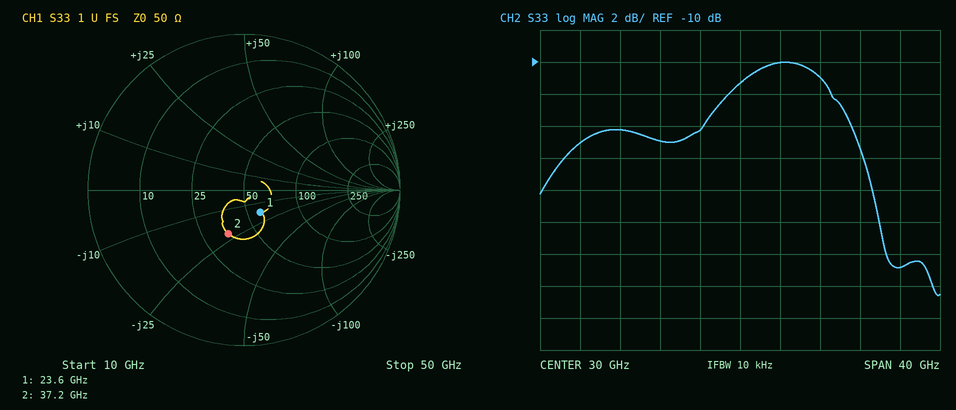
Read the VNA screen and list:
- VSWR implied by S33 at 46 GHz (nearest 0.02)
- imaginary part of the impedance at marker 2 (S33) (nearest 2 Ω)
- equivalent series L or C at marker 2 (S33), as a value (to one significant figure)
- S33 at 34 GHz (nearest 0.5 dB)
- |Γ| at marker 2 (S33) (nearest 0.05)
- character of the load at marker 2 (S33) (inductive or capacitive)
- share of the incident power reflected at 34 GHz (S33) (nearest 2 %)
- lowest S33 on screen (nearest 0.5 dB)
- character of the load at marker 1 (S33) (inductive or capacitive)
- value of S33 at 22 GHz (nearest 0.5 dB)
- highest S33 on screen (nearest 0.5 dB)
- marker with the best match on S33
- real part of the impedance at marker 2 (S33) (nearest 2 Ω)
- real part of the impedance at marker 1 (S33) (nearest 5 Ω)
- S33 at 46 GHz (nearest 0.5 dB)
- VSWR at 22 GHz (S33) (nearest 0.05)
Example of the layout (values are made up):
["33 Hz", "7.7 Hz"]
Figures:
["1.16", "-22 Ω", "200 fF", "-10.0 dB", "0.30", "capacitive", "10 %", "-24.5 dB", "capacitive", "-15.0 dB", "-10.0 dB", "marker 1", "36 Ω", "60 Ω", "-23.0 dB", "1.45"]
